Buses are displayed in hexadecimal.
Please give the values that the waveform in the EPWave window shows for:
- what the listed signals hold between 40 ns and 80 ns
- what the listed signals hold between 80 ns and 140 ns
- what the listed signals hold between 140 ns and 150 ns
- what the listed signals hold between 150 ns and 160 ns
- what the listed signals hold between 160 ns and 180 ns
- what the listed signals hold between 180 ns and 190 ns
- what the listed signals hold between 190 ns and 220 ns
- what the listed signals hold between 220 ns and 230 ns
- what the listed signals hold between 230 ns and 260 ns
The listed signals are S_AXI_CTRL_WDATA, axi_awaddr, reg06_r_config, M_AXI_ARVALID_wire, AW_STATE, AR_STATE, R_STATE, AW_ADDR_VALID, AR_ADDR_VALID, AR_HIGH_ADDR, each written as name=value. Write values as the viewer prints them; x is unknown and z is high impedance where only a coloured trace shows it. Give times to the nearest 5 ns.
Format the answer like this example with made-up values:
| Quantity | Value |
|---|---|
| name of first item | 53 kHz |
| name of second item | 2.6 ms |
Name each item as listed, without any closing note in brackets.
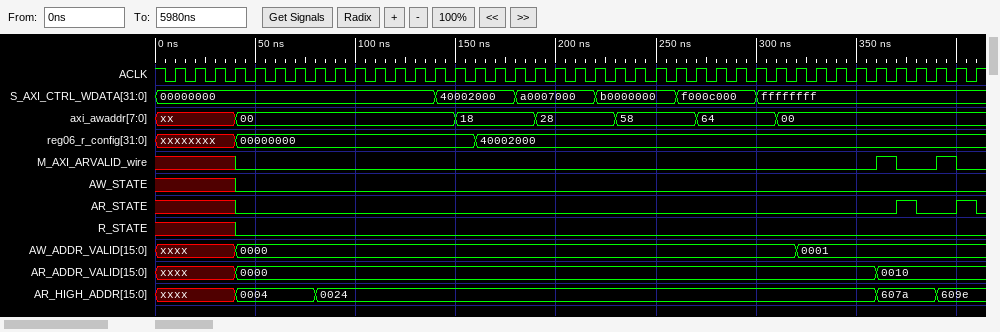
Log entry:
| Quantity | Value |
|---|---|
| what the listed signals hold between 40 ns and 80 ns | S_AXI_CTRL_WDATA=00000000, axi_awaddr=00, reg06_r_config=00000000, M_AXI_ARVALID_wire=0, AW_STATE=0, AR_STATE=0, R_STATE=0, AW_ADDR_VALID=0000, AR_ADDR_VALID=0000, AR_HIGH_ADDR=0004 |
| what the listed signals hold between 80 ns and 140 ns | S_AXI_CTRL_WDATA=00000000, axi_awaddr=00, reg06_r_config=00000000, M_AXI_ARVALID_wire=0, AW_STATE=0, AR_STATE=0, R_STATE=0, AW_ADDR_VALID=0000, AR_ADDR_VALID=0000, AR_HIGH_ADDR=0024 |
| what the listed signals hold between 140 ns and 150 ns | S_AXI_CTRL_WDATA=40002000, axi_awaddr=00, reg06_r_config=00000000, M_AXI_ARVALID_wire=0, AW_STATE=0, AR_STATE=0, R_STATE=0, AW_ADDR_VALID=0000, AR_ADDR_VALID=0000, AR_HIGH_ADDR=0024 |
| what the listed signals hold between 150 ns and 160 ns | S_AXI_CTRL_WDATA=40002000, axi_awaddr=18, reg06_r_config=00000000, M_AXI_ARVALID_wire=0, AW_STATE=0, AR_STATE=0, R_STATE=0, AW_ADDR_VALID=0000, AR_ADDR_VALID=0000, AR_HIGH_ADDR=0024 |
| what the listed signals hold between 160 ns and 180 ns | S_AXI_CTRL_WDATA=40002000, axi_awaddr=18, reg06_r_config=40002000, M_AXI_ARVALID_wire=0, AW_STATE=0, AR_STATE=0, R_STATE=0, AW_ADDR_VALID=0000, AR_ADDR_VALID=0000, AR_HIGH_ADDR=0024 |
| what the listed signals hold between 180 ns and 190 ns | S_AXI_CTRL_WDATA=a0007000, axi_awaddr=18, reg06_r_config=40002000, M_AXI_ARVALID_wire=0, AW_STATE=0, AR_STATE=0, R_STATE=0, AW_ADDR_VALID=0000, AR_ADDR_VALID=0000, AR_HIGH_ADDR=0024 |
| what the listed signals hold between 190 ns and 220 ns | S_AXI_CTRL_WDATA=a0007000, axi_awaddr=28, reg06_r_config=40002000, M_AXI_ARVALID_wire=0, AW_STATE=0, AR_STATE=0, R_STATE=0, AW_ADDR_VALID=0000, AR_ADDR_VALID=0000, AR_HIGH_ADDR=0024 |
| what the listed signals hold between 220 ns and 230 ns | S_AXI_CTRL_WDATA=b0000000, axi_awaddr=28, reg06_r_config=40002000, M_AXI_ARVALID_wire=0, AW_STATE=0, AR_STATE=0, R_STATE=0, AW_ADDR_VALID=0000, AR_ADDR_VALID=0000, AR_HIGH_ADDR=0024 |
| what the listed signals hold between 230 ns and 260 ns | S_AXI_CTRL_WDATA=b0000000, axi_awaddr=58, reg06_r_config=40002000, M_AXI_ARVALID_wire=0, AW_STATE=0, AR_STATE=0, R_STATE=0, AW_ADDR_VALID=0000, AR_ADDR_VALID=0000, AR_HIGH_ADDR=0024 |
